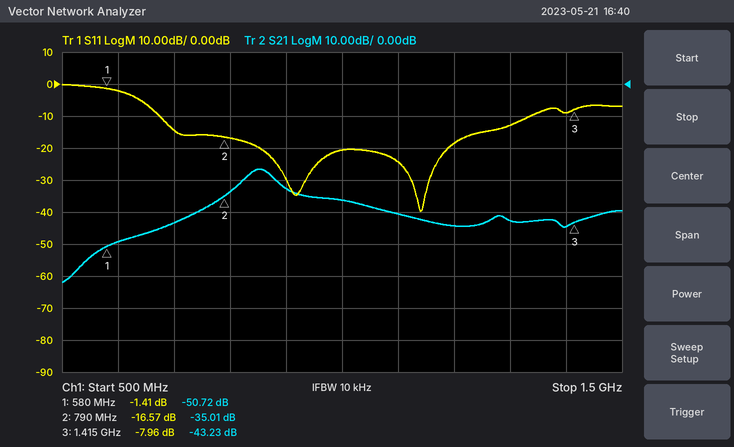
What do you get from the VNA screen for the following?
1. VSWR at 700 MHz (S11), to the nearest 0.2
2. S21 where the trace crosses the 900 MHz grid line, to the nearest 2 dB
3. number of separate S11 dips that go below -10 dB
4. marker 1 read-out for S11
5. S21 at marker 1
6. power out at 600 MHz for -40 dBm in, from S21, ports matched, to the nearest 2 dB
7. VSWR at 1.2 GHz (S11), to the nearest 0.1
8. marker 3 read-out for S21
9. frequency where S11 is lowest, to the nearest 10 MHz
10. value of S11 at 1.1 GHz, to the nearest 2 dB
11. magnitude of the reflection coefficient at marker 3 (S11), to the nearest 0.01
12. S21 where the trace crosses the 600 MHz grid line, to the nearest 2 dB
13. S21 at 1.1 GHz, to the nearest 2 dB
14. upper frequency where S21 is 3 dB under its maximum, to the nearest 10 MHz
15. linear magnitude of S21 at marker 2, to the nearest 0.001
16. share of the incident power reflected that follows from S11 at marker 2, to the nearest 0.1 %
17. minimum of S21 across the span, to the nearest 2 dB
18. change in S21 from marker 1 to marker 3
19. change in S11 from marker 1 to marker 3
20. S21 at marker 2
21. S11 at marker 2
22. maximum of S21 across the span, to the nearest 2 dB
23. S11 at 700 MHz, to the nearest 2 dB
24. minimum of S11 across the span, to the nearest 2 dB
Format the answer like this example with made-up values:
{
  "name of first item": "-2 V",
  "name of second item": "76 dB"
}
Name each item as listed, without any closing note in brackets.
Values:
{
  "VSWR at 700 MHz (S11), to the nearest 0.2": "1.4",
  "S21 where the trace crosses the 900 MHz grid line, to the nearest 2 dB": "-32 dB",
  "number of separate S11 dips that go below -10 dB": "2",
  "marker 1 read-out for S11": "-1.41 dB",
  "S21 at marker 1": "-50.72 dB",
  "power out at 600 MHz for -40 dBm in, from S21, ports matched, to the nearest 2 dB": "-90 dBm",
  "VSWR at 1.2 GHz (S11), to the nearest 0.1": "1.3",
  "marker 3 read-out for S21": "-43.23 dB",
  "frequency where S11 is lowest, to the nearest 10 MHz": "1.14 GHz",
  "value of S11 at 1.1 GHz, to the nearest 2 dB": "-24 dB",
  "magnitude of the reflection coefficient at marker 3 (S11), to the nearest 0.01": "0.40",
  "S21 where the trace crosses the 600 MHz grid line, to the nearest 2 dB": "-50 dB",
  "S21 at 1.1 GHz, to the nearest 2 dB": "-40 dB",
  "upper frequency where S21 is 3 dB under its maximum, to the nearest 10 MHz": "880 MHz",
  "linear magnitude of S21 at marker 2, to the nearest 0.001": "0.018",
  "share of the incident power reflected that follows from S11 at marker 2, to the nearest 0.1 %": "2.2 %",
  "minimum of S21 across the span, to the nearest 2 dB": "-62 dB",
  "change in S21 from marker 1 to marker 3": "7.49 dB",
  "change in S11 from marker 1 to marker 3": "-6.55 dB",
  "S21 at marker 2": "-35.01 dB",
  "S11 at marker 2": "-16.57 dB",
  "maximum of S21 across the span, to the nearest 2 dB": "-26 dB",
  "S11 at 700 MHz, to the nearest 2 dB": "-14 dB",
  "minimum of S11 across the span, to the nearest 2 dB": "-40 dB"
}
